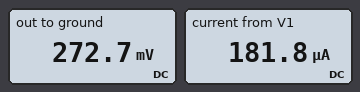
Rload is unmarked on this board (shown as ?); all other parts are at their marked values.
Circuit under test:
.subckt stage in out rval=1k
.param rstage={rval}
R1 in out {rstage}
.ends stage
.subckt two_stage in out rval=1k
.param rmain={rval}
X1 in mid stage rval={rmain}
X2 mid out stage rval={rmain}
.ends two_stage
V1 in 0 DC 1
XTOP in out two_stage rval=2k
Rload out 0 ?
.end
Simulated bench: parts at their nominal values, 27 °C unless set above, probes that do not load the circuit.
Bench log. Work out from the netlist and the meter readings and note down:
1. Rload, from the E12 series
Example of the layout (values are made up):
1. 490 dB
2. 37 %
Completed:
1. 1.5 kΩ
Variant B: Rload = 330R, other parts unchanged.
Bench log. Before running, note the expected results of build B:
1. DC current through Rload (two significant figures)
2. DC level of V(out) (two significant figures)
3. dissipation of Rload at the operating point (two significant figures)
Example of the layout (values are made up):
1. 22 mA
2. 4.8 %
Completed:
1. 230 µA
2. 76 mV
3. 18 µW
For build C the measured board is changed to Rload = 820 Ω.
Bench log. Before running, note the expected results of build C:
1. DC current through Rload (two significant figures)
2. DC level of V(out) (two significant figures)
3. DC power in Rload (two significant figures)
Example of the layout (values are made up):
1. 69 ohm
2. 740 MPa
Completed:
1. 210 µA
2. 170 mV
3. 35 µW
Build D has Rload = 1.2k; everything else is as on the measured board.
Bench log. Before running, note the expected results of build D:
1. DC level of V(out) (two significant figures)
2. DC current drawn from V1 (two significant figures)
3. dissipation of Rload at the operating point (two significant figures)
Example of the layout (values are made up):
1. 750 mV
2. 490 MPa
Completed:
1. 230 mV
2. 190 µA
3. 44 µW
